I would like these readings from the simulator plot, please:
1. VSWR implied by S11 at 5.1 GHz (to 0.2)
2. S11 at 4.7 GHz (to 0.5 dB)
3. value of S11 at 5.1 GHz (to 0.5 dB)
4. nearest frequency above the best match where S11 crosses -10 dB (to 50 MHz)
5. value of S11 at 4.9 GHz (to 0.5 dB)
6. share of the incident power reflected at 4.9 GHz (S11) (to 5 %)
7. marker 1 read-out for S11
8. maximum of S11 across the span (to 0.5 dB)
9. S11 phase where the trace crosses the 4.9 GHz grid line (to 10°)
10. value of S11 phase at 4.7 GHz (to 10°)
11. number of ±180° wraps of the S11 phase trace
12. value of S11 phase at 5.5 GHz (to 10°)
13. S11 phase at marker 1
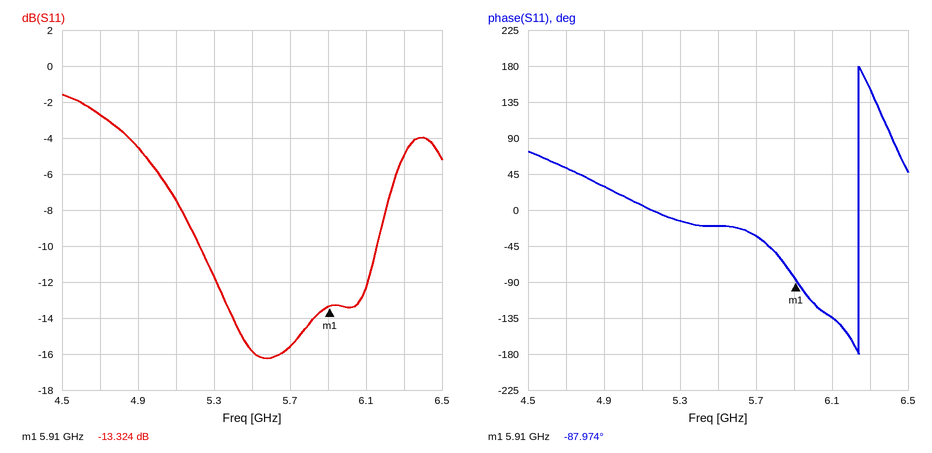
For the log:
2.4
-2.5 dB
-7.5 dB
6.15 GHz
-4.5 dB
35 %
-13.324 dB
-1.5 dB
30°
50°
1
-20°
-87.974°
